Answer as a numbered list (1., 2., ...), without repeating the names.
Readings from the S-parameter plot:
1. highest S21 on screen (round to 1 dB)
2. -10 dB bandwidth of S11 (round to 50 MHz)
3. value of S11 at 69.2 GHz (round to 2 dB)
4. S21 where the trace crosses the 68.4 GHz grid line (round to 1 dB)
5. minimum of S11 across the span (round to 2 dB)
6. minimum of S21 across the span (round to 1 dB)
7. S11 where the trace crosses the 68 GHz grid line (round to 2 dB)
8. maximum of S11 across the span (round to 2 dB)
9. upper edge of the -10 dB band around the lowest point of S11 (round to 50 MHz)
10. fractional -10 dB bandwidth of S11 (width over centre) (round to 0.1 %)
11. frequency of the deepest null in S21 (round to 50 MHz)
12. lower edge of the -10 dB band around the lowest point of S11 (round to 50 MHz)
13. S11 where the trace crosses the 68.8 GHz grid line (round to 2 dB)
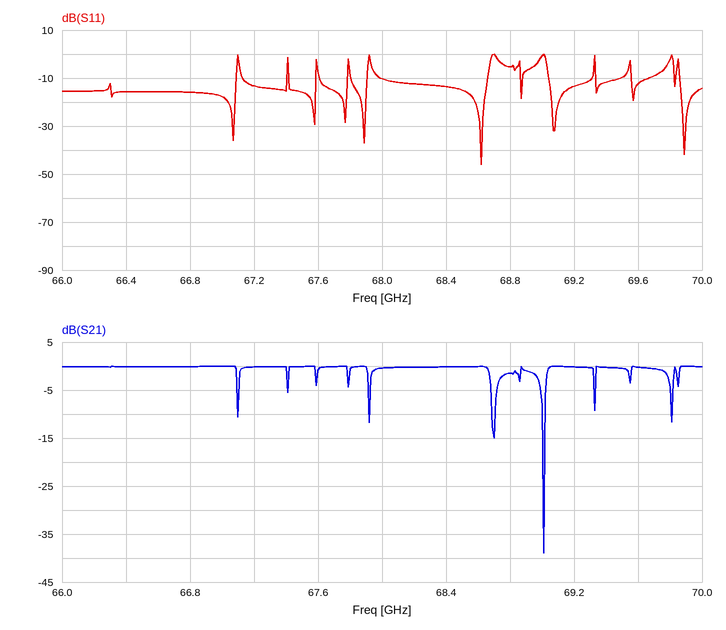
1. 0 dB
2. 650 MHz
3. -14 dB
4. 0 dB
5. -46 dB
6. -39 dB
7. -10 dB
8. 0 dB
9. 68.65 GHz
10. 1.0 %
11. 69.00 GHz
12. 68.00 GHz
13. -6 dB
